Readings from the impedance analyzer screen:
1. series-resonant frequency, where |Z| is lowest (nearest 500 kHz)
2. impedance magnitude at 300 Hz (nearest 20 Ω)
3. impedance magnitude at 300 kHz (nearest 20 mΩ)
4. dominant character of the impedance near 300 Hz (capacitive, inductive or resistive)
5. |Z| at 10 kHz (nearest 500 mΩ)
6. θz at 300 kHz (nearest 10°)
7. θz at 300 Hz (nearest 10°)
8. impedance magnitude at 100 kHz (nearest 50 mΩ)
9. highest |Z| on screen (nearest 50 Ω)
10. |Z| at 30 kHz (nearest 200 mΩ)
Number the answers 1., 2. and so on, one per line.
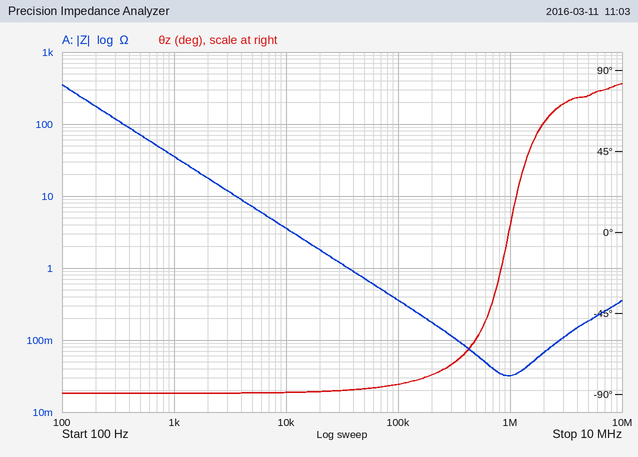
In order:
1. 1.0 MHz
2. 120 Ω
3. 120 mΩ
4. capacitive
5. 3.5 Ω
6. -70°
7. -90°
8. 350 mΩ
9. 350 Ω
10. 1.2 Ω
